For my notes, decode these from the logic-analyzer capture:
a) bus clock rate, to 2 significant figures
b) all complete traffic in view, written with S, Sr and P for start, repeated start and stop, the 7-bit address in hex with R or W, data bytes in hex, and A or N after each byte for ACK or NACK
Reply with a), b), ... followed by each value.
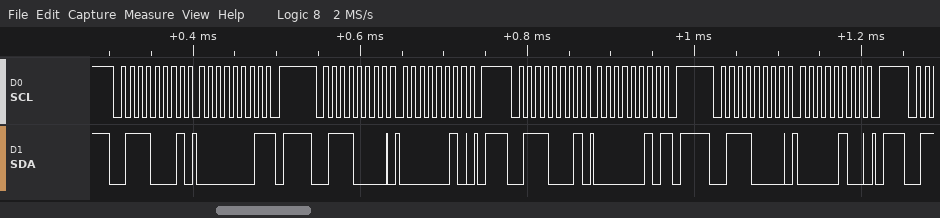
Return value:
a) 100 kHz
b) S 38R A 01 N P S 38W A 02 A P S 38R A 02 N P S 38W A 04 A P
